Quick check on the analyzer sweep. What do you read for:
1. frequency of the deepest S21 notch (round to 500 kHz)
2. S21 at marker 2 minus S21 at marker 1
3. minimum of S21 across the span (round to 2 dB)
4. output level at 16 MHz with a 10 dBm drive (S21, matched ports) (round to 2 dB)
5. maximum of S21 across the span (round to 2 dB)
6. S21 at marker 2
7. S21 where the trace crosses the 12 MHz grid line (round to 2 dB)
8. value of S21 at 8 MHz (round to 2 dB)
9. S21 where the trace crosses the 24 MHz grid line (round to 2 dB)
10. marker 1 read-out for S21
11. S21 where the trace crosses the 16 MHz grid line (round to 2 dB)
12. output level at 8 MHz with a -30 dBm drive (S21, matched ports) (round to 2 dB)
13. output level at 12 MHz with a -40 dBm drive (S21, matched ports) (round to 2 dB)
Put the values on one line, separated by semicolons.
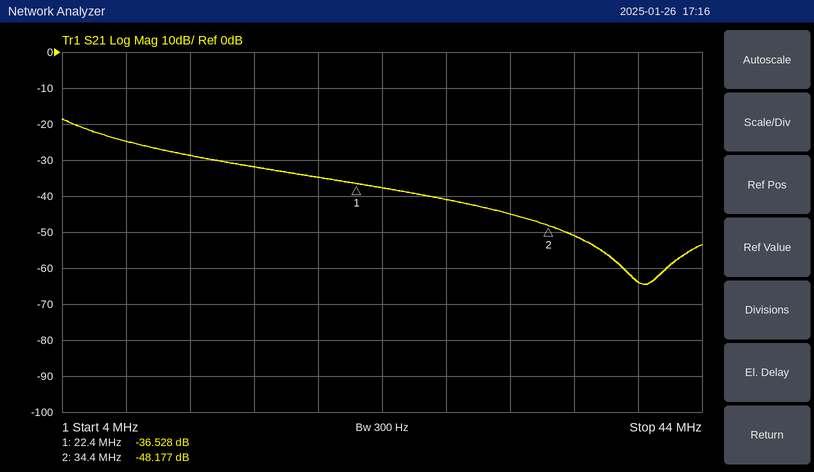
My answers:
40.5 MHz; -11.649 dB; -64 dB; -22 dBm; -18 dB; -48.177 dB; -28 dB; -24 dB; -38 dB; -36.528 dB; -32 dB; -54 dBm; -68 dBm
